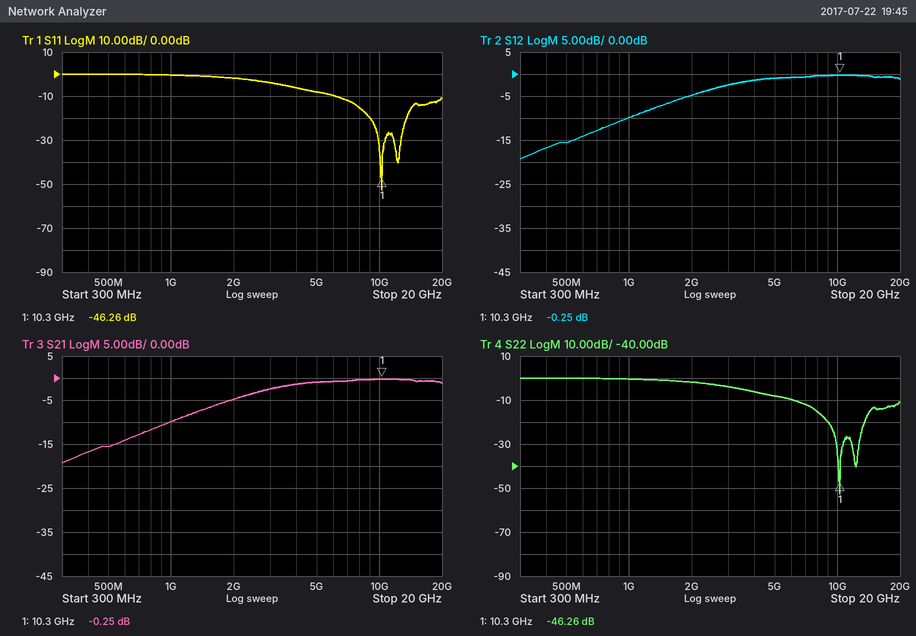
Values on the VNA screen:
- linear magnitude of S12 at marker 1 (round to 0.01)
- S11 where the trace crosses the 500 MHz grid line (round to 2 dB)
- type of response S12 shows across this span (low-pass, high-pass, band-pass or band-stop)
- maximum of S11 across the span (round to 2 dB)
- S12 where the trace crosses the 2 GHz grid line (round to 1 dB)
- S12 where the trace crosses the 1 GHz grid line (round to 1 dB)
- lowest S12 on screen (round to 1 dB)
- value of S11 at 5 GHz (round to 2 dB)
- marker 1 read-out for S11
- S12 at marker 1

0.97
0 dB
high-pass
0 dB
-5 dB
-10 dB
-19 dB
-8 dB
-46.26 dB
-0.25 dB
